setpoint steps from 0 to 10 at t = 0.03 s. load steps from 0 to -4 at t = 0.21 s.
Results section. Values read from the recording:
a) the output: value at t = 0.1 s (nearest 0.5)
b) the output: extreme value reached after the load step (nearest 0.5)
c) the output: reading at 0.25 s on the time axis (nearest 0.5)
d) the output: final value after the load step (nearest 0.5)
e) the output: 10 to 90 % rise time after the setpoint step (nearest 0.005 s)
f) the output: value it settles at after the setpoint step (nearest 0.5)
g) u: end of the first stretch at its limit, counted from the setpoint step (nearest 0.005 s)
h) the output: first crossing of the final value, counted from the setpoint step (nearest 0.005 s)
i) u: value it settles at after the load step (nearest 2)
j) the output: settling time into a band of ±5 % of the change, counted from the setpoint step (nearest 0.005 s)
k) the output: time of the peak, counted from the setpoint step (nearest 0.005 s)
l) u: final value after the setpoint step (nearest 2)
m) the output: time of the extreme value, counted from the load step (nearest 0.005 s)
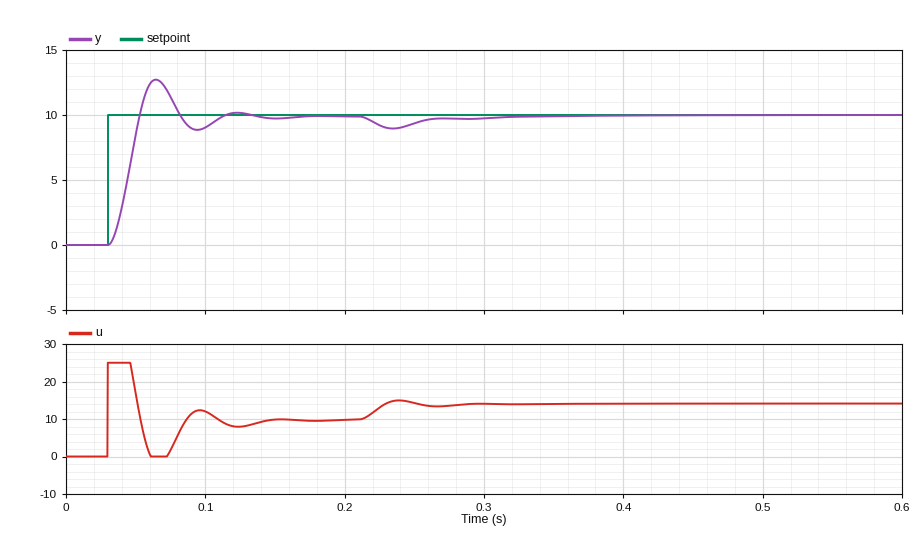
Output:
9.0
9.0
9.5
10.0
0.015 s
10.0
0.015 s
0.025 s
14
0.075 s
0.035 s
10
0.025 s
